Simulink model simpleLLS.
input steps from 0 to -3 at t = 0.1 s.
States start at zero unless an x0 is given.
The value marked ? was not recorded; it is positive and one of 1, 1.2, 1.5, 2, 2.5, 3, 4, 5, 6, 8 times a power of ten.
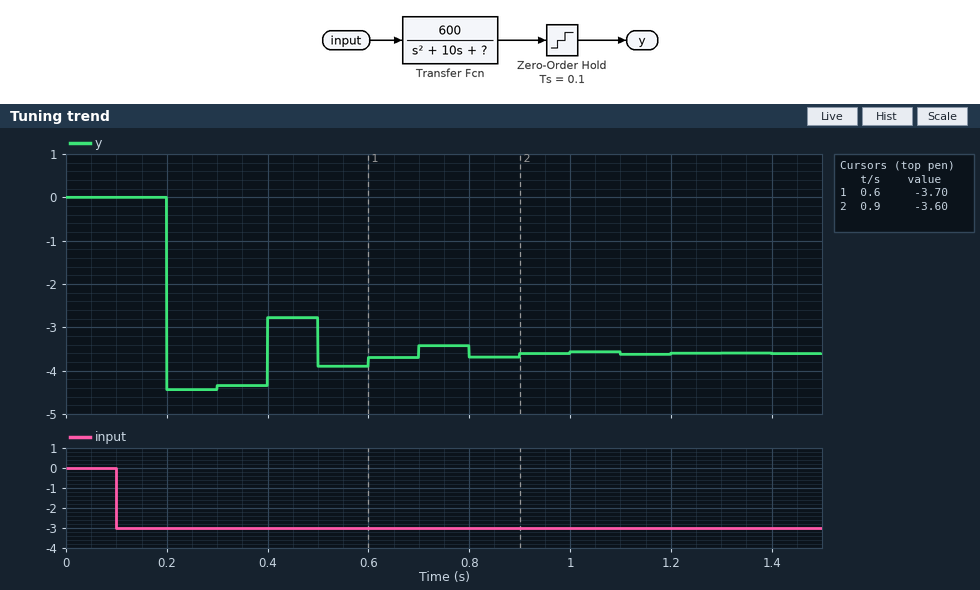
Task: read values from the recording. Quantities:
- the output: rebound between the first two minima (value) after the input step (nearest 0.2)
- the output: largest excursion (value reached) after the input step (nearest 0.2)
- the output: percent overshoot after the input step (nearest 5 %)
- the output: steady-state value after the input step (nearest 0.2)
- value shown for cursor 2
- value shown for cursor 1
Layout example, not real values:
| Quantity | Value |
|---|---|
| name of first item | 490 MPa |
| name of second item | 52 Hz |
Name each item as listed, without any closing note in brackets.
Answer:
| Quantity | Value |
|---|---|
| the output: rebound between the first two minima (value) after the input step | -2.8 |
| the output: largest excursion (value reached) after the input step | -4.4 |
| the output: percent overshoot after the input step | 25 % |
| the output: steady-state value after the input step | -3.6 |
| value shown for cursor 2 | -3.60 |
| value shown for cursor 1 | -3.70 |
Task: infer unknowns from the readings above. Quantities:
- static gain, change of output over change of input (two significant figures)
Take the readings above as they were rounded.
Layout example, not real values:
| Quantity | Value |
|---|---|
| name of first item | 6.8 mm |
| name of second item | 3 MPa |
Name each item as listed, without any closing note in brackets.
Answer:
| Quantity | Value |
|---|---|
| static gain, change of output over change of input | 1.2 |
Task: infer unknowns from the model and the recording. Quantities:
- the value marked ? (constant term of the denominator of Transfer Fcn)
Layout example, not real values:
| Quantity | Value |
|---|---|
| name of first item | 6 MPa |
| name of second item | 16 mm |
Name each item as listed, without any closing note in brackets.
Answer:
| Quantity | Value |
|---|---|
| the value marked ? | 500 |
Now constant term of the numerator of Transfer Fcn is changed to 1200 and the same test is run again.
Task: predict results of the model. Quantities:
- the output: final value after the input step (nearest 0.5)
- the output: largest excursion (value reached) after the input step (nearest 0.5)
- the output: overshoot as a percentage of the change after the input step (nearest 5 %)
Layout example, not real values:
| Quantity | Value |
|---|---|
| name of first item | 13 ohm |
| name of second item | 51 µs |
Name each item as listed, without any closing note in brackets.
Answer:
| Quantity | Value |
|---|---|
| the output: final value after the input step | -7.0 |
| the output: largest excursion (value reached) after the input step | -9.0 |
| the output: overshoot as a percentage of the change after the input step | 25 % |
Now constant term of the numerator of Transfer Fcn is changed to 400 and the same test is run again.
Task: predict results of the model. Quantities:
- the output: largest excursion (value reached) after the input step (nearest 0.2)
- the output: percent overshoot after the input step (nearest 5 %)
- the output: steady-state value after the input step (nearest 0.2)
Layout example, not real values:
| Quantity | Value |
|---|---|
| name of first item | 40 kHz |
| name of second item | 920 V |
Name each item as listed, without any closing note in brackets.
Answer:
| Quantity | Value |
|---|---|
| the output: largest excursion (value reached) after the input step | -3.0 |
| the output: percent overshoot after the input step | 25 % |
| the output: steady-state value after the input step | -2.4 |
